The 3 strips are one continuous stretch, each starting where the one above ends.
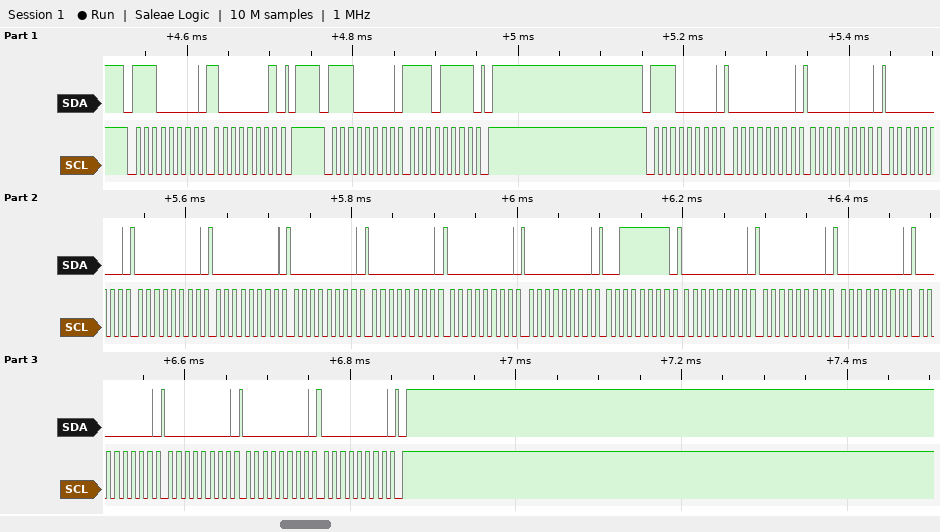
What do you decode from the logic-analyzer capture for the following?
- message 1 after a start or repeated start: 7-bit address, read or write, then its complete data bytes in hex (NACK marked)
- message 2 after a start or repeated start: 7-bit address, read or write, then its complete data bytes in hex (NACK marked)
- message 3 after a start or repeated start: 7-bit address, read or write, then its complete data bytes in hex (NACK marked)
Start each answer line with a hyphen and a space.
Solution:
- 0x70 write: 81
- 0x70 write: EF
- 0x70 write: 00 00 00 00 00 00 00 00 00 3F 00 00 00 00 00 00 00
